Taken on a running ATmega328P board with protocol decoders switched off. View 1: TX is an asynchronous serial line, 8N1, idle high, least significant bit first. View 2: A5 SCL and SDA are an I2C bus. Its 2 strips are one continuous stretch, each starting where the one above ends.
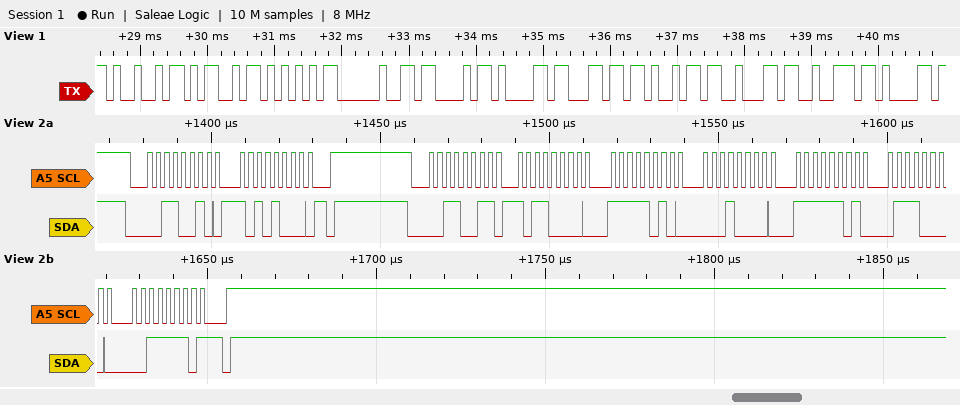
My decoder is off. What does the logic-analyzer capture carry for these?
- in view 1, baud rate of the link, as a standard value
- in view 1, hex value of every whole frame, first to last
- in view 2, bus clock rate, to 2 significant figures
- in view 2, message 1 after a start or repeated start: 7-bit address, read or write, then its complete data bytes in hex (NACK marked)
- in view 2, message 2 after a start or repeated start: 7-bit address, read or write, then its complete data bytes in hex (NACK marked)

9600 baud
49 4D 55 20 43 61 6C 69 62 72 61
400 kHz
0x19 write: A8
0x19 read: B0 FA 10 FD 70 3E NACK
